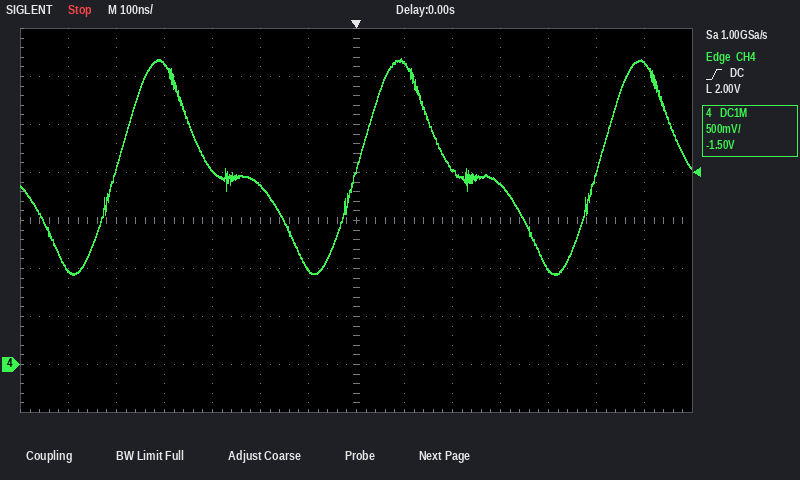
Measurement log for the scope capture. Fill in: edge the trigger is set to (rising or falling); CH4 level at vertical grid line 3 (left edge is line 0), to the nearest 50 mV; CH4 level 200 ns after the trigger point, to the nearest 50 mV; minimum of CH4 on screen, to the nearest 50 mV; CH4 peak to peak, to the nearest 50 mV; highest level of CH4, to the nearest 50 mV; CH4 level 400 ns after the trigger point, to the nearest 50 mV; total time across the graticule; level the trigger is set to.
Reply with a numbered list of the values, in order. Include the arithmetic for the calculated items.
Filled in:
1. rising
2. 3.15 V
3. 2.05 V
4. 950 mV
5. 3.20 V − (950 mV) = 2.25 V
6. 3.20 V
7. 1.00 V
8. 1.4 µs
9. 2.00 V
